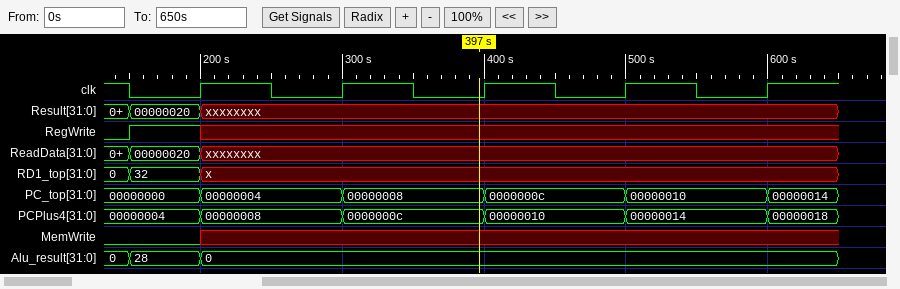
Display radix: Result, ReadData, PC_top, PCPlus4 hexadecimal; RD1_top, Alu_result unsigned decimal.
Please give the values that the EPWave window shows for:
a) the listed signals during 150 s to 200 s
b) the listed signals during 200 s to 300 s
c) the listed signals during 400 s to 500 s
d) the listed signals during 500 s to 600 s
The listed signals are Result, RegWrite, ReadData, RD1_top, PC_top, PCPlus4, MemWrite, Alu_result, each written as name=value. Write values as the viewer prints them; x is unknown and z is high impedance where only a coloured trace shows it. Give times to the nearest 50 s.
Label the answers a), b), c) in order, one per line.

a) Result=00000020, RegWrite=1, ReadData=00000020, RD1_top=32, PC_top=00000000, PCPlus4=00000004, MemWrite=0, Alu_result=28
b) Result=xxxxxxxx, RegWrite=x, ReadData=xxxxxxxx, RD1_top=x, PC_top=00000004, PCPlus4=00000008, MemWrite=x, Alu_result=0
c) Result=xxxxxxxx, RegWrite=x, ReadData=xxxxxxxx, RD1_top=x, PC_top=0000000c, PCPlus4=00000010, MemWrite=x, Alu_result=0
d) Result=xxxxxxxx, RegWrite=x, ReadData=xxxxxxxx, RD1_top=x, PC_top=00000010, PCPlus4=00000014, MemWrite=x, Alu_result=0
